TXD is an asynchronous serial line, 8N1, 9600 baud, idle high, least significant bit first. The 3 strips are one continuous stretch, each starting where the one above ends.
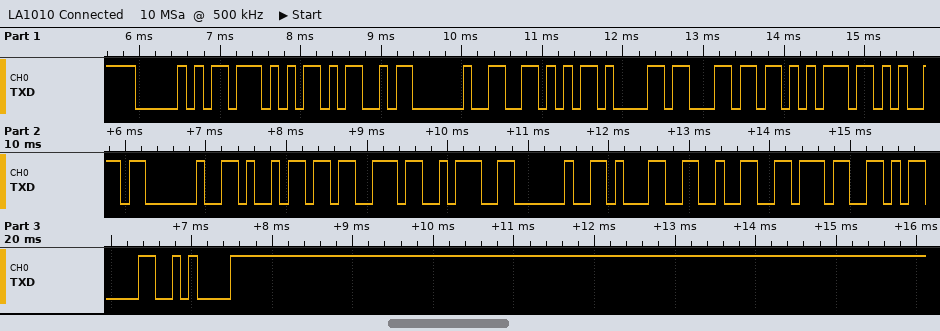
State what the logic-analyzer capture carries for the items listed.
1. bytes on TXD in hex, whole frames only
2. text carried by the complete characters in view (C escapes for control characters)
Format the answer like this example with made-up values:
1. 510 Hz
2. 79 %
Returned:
1. 50 57 4D 20 56 61 6C 75 65 20 69 73 3A 20 31 32 37 0D 0A
2. "PWM Value is: 127\r\n"
